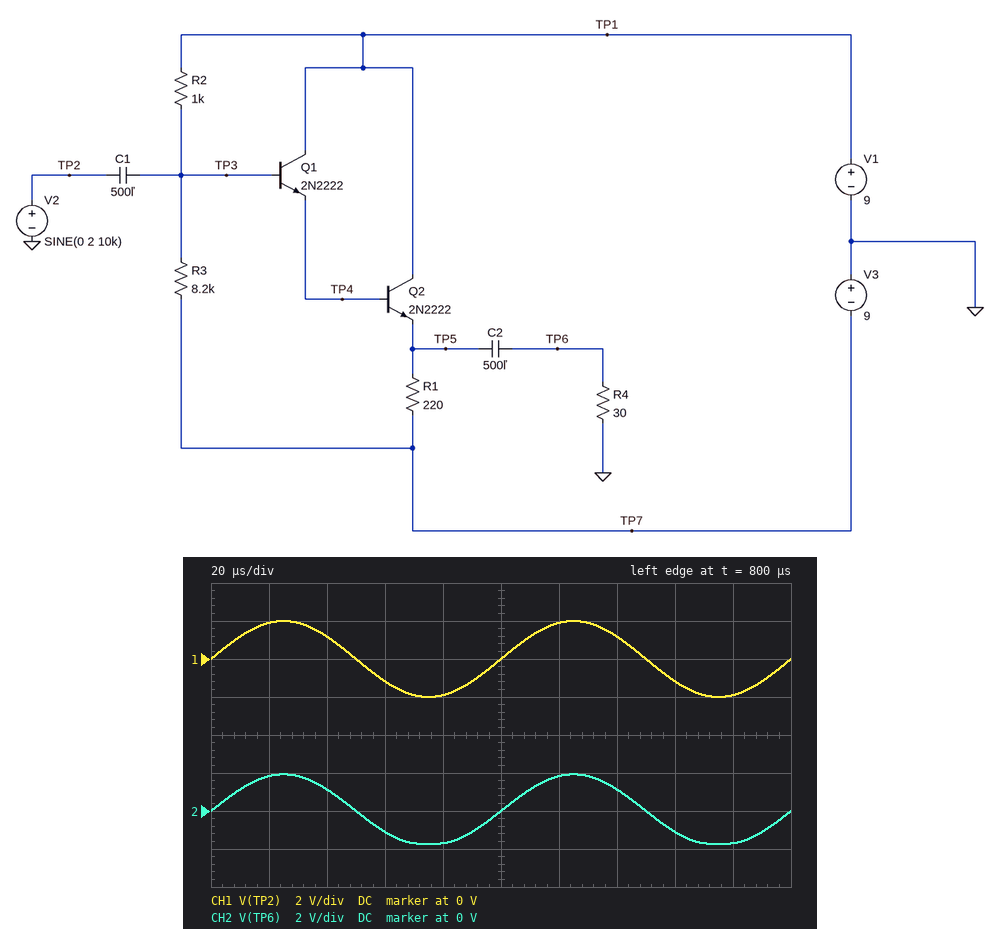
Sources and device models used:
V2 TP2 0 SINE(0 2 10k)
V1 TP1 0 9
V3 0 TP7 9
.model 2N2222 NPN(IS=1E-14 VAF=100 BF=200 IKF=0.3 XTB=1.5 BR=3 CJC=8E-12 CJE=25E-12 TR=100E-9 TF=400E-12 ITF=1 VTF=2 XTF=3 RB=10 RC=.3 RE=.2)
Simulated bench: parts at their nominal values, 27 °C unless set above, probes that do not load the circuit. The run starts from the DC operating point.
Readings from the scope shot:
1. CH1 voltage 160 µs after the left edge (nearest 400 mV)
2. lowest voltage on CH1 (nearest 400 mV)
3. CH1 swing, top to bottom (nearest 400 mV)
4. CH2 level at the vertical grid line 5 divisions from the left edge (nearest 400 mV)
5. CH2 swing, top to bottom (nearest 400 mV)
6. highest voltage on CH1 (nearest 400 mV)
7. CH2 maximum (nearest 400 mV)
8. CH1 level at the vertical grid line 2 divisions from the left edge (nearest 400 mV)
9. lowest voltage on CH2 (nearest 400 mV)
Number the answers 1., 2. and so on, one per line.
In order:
1. -1.2 V
2. -2.0 V
3. 4.0 V
4. 0 V
5. 3.6 V
6. 2.0 V
7. 2.0 V
8. 1.2 V
9. -1.6 V
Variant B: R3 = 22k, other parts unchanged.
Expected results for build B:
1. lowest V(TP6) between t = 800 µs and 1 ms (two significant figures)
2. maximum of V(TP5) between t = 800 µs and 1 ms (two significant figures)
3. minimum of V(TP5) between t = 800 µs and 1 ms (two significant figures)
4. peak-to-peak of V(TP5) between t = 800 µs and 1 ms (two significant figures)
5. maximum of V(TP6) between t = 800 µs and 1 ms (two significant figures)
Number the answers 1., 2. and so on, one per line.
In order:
1. -1.8 V
2. 8.2 V
3. 5.0 V
4. 3.2 V
5. 1.4 V
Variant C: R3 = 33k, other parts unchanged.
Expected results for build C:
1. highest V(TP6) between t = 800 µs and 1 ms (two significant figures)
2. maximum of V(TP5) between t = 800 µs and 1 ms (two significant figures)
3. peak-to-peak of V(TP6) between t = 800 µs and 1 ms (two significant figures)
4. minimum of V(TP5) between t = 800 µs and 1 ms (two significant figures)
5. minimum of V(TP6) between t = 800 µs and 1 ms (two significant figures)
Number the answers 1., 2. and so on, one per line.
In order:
1. 1.2 V
2. 8.2 V
3. 3.0 V
4. 5.2 V
5. -1.8 V
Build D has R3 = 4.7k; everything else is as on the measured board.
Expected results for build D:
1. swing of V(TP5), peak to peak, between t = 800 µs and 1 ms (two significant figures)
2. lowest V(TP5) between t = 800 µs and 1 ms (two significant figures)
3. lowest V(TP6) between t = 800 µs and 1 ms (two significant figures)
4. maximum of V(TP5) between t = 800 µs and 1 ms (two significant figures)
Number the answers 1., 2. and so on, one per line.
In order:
1. 3.5 V
2. 2.8 V
3. -1.6 V
4. 6.4 V
